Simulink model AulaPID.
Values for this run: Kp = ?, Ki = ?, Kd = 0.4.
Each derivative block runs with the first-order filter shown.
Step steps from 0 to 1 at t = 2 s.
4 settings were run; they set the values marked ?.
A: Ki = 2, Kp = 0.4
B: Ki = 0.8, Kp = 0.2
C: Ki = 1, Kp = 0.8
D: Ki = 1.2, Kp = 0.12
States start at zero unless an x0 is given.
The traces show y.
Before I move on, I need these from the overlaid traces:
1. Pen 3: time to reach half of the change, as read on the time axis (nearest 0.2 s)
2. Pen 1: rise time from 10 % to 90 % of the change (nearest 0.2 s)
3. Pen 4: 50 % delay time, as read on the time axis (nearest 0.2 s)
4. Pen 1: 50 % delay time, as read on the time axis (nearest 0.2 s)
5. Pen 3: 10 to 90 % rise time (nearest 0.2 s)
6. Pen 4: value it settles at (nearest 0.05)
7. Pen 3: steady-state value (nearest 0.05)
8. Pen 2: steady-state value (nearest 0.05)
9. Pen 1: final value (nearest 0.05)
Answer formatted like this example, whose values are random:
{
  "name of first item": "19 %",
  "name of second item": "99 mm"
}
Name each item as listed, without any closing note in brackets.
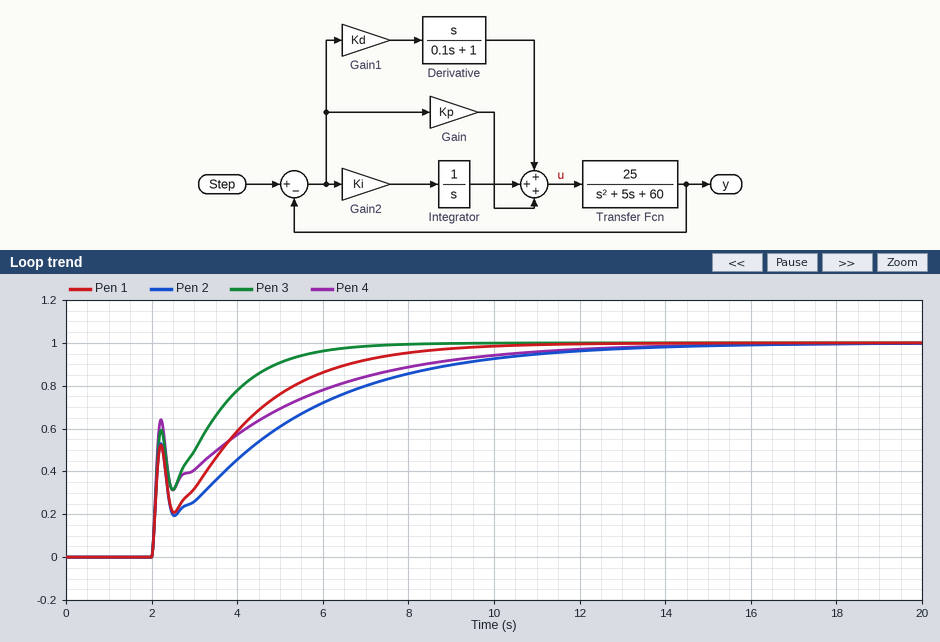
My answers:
{
  "Pen 3: time to reach half of the change, as read on the time axis": "2.2 s",
  "Pen 1: rise time from 10 % to 90 % of the change": "4.6 s",
  "Pen 4: 50 % delay time, as read on the time axis": "2.2 s",
  "Pen 1: 50 % delay time, as read on the time axis": "2.2 s",
  "Pen 3: 10 to 90 % rise time": "2.8 s",
  "Pen 4: value it settles at": "1.00",
  "Pen 3: steady-state value": "1.00",
  "Pen 2: steady-state value": "1.00",
  "Pen 1: final value": "1.00"
}
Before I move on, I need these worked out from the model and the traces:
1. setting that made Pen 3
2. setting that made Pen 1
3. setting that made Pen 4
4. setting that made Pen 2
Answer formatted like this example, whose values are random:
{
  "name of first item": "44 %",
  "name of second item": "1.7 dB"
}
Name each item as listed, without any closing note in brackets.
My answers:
{
  "setting that made Pen 3": "A",
  "setting that made Pen 1": "D",
  "setting that made Pen 4": "C",
  "setting that made Pen 2": "B"
}
